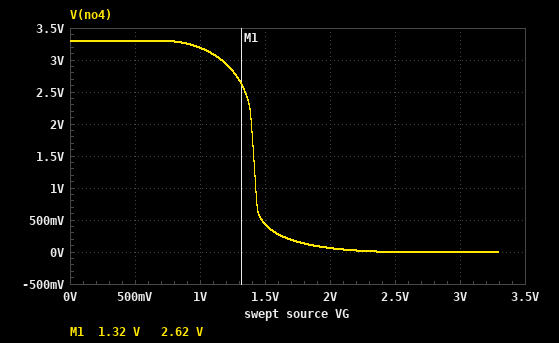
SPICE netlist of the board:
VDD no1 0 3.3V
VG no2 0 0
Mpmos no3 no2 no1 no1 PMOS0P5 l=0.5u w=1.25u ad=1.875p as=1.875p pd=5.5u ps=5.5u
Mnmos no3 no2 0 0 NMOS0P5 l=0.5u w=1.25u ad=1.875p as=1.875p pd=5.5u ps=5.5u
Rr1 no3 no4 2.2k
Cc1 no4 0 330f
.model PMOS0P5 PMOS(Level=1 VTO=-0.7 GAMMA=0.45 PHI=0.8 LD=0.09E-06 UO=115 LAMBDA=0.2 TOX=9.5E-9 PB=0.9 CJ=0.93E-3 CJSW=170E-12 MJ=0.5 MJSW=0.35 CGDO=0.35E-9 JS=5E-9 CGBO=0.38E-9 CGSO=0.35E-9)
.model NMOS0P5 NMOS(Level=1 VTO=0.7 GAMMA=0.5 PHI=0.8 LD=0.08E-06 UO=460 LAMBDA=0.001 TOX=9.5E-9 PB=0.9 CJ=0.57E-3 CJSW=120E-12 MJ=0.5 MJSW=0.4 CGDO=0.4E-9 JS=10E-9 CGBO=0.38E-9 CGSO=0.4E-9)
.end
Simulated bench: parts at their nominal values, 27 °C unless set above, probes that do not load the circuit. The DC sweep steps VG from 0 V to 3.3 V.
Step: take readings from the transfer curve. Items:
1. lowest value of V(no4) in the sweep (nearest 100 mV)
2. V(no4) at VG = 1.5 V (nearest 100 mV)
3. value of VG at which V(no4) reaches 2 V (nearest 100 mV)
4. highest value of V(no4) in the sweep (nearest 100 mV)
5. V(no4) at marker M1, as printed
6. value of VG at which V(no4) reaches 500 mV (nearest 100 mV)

0 V
400 mV
1.4 V
3.3 V
2.62 V
1.5 V
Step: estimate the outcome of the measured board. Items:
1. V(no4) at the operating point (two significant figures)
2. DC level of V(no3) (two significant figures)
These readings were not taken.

3.3 V
3.3 V
